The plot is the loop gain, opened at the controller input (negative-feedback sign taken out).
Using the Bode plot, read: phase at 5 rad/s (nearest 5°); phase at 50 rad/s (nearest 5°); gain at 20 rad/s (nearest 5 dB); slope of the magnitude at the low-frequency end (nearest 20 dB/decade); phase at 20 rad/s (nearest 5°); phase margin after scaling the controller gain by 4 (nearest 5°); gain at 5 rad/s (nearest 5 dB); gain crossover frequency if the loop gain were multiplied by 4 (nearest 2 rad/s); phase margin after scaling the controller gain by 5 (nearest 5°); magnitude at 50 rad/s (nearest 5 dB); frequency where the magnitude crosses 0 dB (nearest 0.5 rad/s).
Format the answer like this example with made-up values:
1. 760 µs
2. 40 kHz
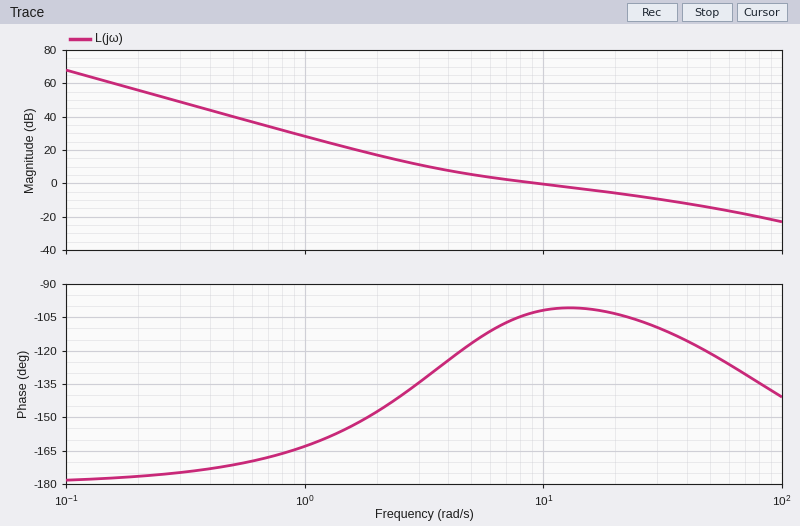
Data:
1. -115°
2. -120°
3. -5 dB
4. -40 dB/decade
5. -105°
6. 65°
7. 5 dB
8. 40 rad/s
9. 60°
10. -15 dB
11. 9.5 rad/s
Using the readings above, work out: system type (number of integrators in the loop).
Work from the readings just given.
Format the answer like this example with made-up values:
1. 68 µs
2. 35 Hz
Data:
1. 2
